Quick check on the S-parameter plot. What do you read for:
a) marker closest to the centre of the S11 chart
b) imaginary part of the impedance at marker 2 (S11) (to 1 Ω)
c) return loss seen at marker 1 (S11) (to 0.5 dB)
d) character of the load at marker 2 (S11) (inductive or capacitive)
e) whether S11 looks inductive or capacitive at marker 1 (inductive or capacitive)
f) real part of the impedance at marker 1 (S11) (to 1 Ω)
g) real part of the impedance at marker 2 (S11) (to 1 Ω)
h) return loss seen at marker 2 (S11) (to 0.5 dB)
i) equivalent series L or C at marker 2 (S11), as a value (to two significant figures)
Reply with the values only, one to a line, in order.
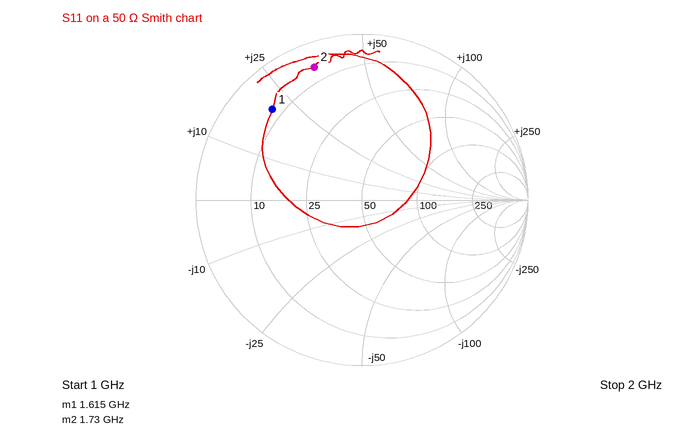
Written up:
marker 1
+35 Ω
2.5 dB
inductive
inductive
8 Ω
6 Ω
1.5 dB
3.2 nH
